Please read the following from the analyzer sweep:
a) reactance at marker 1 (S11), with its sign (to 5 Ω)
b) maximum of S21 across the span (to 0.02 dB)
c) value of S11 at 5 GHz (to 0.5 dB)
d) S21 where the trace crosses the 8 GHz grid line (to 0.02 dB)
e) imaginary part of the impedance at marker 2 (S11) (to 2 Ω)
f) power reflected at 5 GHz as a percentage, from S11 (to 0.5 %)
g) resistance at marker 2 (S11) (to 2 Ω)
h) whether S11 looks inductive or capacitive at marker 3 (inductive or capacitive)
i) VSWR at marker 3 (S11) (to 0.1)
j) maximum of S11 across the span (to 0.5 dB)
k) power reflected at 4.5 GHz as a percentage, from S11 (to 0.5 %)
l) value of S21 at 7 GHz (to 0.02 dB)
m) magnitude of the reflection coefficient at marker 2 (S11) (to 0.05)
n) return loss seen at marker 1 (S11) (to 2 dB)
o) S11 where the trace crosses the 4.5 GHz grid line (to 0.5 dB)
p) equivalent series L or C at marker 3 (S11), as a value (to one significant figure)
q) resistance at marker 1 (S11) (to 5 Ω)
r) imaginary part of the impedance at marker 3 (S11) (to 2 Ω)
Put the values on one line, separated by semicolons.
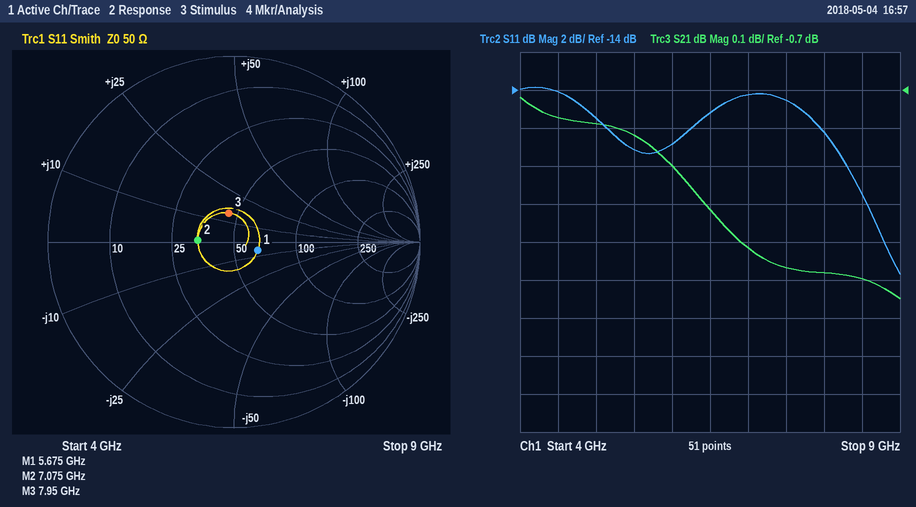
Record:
-5 Ω; -0.72 dB; -15.5 dB; -1.18 dB; 0 Ω; 3.0 %; 34 Ω; inductive; 1.4; -14.0 dB; 4.0 %; -1.12 dB; 0.20; 18 dB; -14.0 dB; 300 pH; 65 Ω; +14 Ω
